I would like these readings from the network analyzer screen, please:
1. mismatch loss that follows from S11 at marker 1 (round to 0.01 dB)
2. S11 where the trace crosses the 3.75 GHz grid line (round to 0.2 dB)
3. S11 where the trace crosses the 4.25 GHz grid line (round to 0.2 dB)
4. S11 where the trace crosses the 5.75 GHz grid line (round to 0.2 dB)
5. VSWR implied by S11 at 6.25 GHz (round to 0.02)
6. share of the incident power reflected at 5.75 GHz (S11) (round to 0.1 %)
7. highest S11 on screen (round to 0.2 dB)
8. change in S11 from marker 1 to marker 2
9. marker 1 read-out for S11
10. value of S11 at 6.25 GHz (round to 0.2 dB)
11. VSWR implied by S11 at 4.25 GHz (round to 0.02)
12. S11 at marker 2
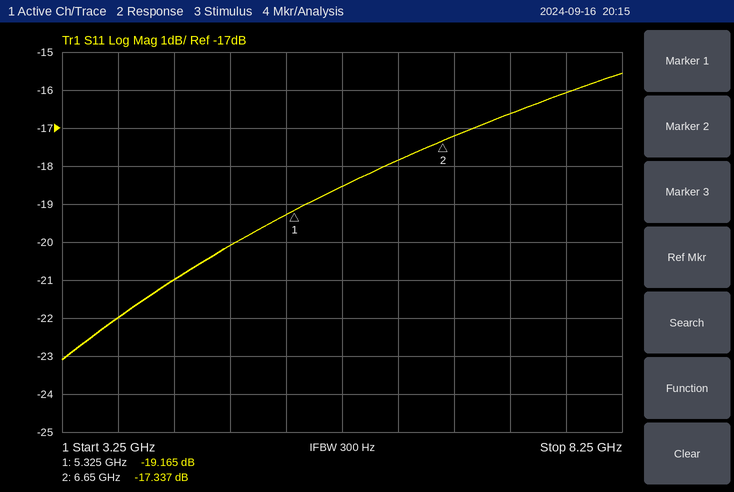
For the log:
0.05 dB
-22.0 dB
-21.0 dB
-18.6 dB
1.30
1.4 %
-15.6 dB
1.828 dB
-19.165 dB
-17.8 dB
1.20
-17.337 dB
